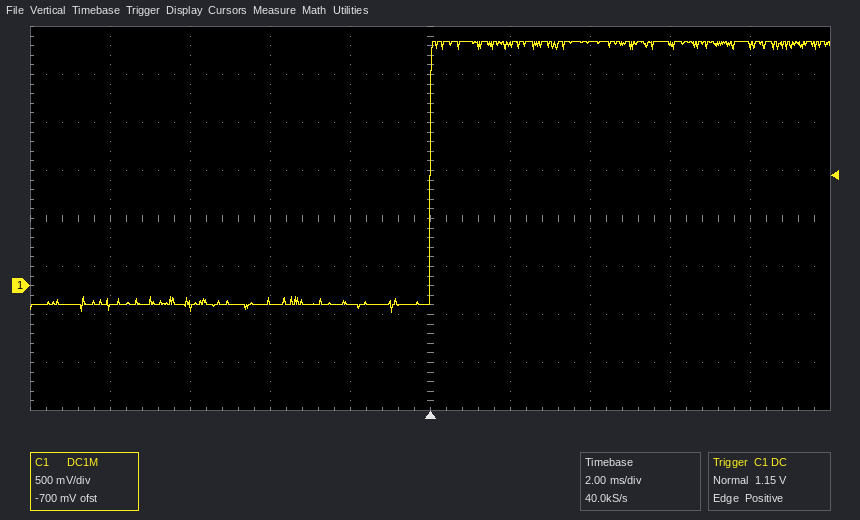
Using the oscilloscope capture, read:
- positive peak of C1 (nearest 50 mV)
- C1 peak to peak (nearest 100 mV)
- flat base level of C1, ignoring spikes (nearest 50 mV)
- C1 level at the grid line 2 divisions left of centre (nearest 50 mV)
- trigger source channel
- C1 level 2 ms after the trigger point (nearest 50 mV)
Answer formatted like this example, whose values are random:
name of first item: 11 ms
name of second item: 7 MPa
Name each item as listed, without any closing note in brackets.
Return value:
positive peak of C1: 2.55 V
C1 peak to peak: 2.80 V
flat base level of C1, ignoring spikes: -200 mV
C1 level at the grid line 2 divisions left of centre: -150 mV
trigger source channel: C1
C1 level 2 ms after the trigger point: 2.50 V
